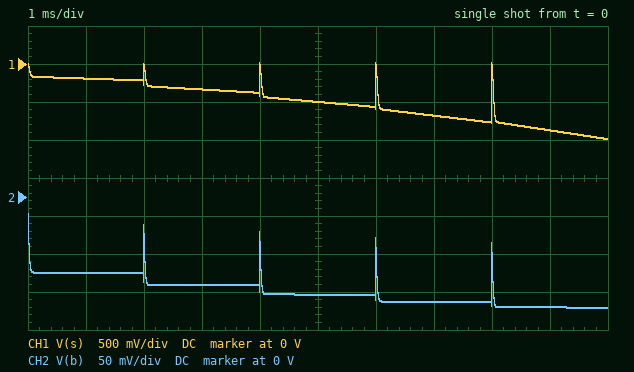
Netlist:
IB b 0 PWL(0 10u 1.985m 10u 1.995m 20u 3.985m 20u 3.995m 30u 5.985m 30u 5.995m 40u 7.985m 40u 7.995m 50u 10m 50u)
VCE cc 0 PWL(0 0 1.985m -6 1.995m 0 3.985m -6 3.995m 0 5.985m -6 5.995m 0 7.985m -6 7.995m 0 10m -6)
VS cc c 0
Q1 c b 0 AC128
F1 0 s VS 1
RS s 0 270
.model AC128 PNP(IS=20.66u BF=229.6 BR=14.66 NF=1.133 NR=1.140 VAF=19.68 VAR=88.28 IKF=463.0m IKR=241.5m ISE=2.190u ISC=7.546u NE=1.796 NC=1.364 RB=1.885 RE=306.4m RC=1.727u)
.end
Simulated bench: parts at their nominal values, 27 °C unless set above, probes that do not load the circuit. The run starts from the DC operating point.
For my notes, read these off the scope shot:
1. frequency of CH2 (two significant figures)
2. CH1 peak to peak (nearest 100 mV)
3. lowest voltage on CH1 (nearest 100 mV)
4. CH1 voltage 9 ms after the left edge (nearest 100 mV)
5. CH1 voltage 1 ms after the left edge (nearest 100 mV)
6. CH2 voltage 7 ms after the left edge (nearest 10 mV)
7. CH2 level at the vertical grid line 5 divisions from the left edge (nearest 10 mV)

500 Hz
1.0 V
-1.0 V
-900 mV
-200 mV
-140 mV
-130 mV
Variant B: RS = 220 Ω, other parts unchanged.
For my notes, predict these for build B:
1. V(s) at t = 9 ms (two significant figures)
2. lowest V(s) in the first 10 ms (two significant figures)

-710 mV
-810 mV
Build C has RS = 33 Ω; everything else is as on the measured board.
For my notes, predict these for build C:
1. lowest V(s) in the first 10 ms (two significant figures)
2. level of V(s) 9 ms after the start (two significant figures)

-120 mV
-110 mV
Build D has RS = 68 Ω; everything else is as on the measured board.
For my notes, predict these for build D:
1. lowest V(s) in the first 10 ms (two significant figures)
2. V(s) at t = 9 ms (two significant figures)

-250 mV
-220 mV
